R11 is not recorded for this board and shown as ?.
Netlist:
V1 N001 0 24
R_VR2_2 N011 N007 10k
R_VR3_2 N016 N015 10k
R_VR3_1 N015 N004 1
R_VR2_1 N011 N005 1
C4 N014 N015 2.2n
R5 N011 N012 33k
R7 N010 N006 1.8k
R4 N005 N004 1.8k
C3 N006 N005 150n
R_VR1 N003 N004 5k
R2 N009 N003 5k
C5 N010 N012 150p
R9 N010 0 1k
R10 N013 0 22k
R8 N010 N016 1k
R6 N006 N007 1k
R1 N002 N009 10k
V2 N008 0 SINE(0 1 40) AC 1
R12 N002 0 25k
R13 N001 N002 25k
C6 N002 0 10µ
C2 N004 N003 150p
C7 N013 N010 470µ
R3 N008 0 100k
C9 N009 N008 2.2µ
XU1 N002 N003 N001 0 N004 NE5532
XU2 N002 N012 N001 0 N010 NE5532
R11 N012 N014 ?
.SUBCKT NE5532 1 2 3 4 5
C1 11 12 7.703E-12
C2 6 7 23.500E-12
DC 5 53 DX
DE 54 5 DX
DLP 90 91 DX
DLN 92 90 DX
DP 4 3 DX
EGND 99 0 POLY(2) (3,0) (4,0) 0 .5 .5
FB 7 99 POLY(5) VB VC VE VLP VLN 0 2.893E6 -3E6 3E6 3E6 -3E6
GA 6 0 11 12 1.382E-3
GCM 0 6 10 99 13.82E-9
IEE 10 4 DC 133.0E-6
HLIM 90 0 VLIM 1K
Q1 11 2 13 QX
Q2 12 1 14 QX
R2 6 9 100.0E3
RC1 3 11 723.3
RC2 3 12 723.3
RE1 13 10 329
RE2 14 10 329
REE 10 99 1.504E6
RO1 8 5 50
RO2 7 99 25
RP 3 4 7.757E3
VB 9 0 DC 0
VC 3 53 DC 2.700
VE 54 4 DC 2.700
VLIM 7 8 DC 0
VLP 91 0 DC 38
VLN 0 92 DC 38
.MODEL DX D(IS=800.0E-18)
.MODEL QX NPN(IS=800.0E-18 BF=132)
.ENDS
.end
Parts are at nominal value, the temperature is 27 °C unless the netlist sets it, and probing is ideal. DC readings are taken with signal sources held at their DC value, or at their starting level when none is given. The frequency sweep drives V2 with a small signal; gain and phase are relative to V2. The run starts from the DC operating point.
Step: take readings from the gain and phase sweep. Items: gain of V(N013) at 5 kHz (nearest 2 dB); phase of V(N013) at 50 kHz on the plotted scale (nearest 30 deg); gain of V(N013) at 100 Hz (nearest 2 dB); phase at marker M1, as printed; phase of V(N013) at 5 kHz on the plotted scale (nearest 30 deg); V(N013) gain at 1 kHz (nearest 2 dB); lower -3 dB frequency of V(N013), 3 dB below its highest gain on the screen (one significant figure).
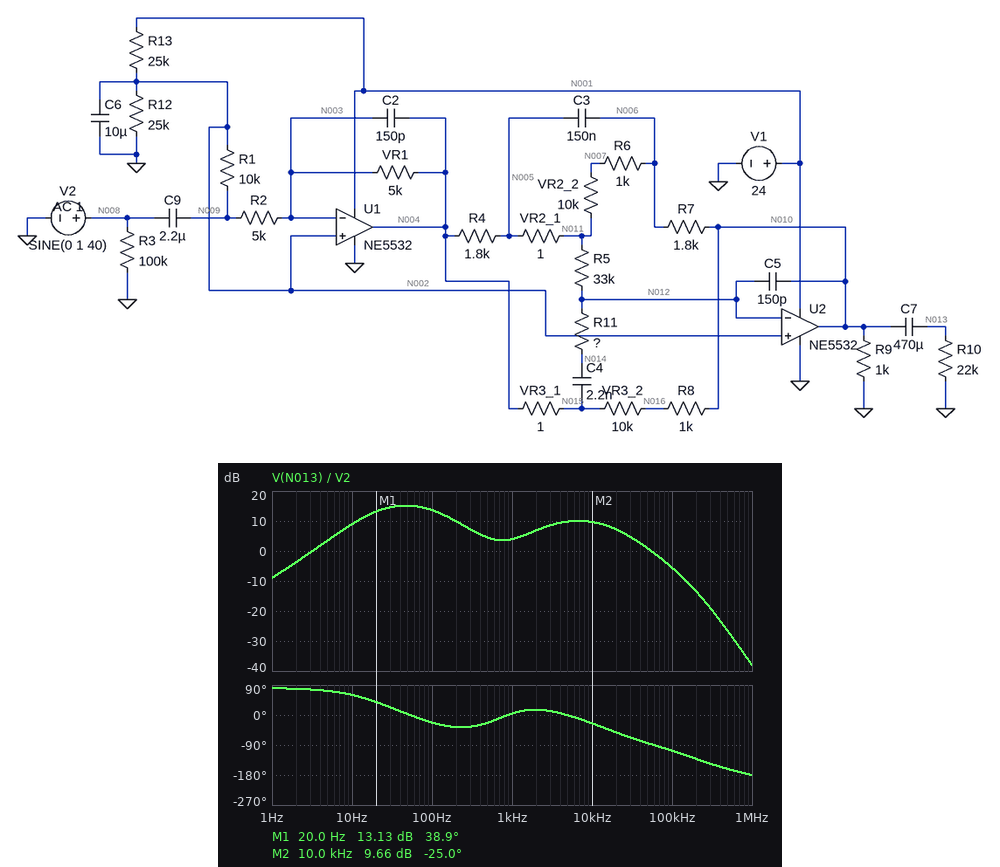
10 dB
-90 deg
14 dB
38.9 deg
0 deg
4 dB
20 Hz
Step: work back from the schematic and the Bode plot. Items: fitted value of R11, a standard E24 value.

24 kΩ
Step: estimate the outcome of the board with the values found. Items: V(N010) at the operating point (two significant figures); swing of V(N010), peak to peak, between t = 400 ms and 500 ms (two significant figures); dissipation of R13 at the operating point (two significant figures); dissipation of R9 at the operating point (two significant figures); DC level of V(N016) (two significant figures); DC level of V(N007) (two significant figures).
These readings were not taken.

12 V
11 V
5.8 mW
150 mW
12 V
12 V
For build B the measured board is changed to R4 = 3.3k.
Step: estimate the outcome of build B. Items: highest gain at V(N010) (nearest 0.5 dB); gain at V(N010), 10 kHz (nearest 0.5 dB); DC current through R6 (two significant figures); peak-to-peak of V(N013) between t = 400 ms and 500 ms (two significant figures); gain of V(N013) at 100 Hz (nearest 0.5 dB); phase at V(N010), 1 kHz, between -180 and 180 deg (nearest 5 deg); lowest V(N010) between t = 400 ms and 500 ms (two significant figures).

10.0 dB
7.5 dB
4.7 µA
6.2 V
8.5 dB
15 deg
9.0 V
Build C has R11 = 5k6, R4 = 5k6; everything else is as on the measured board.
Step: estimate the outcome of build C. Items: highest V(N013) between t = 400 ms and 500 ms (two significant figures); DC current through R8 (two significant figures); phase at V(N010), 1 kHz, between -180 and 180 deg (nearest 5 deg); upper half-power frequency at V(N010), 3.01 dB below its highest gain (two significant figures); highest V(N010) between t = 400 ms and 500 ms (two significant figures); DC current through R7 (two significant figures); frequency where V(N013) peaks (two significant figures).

1.8 V
4.7 µA
40 deg
42 kHz
14 V
3.0 µA
17 kHz
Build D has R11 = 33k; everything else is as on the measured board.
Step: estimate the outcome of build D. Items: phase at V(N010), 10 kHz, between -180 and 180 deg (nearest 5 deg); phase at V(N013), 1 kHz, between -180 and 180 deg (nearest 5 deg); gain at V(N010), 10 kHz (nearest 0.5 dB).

-30 deg
0 deg
8.0 dB
